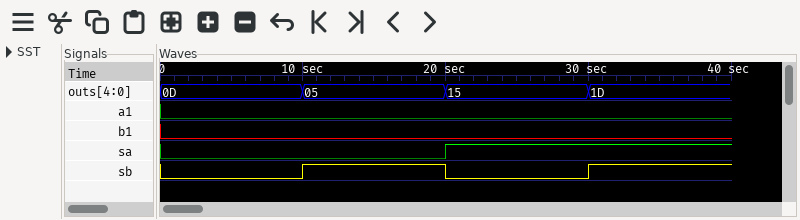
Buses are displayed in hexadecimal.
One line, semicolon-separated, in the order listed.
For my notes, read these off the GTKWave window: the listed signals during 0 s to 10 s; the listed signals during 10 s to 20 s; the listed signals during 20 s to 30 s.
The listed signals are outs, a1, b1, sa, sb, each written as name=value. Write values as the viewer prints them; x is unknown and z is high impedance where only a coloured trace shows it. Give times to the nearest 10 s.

outs=0D, a1=0, b1=0, sa=0, sb=0; outs=05, a1=0, b1=0, sa=0, sb=1; outs=15, a1=0, b1=0, sa=1, sb=0
